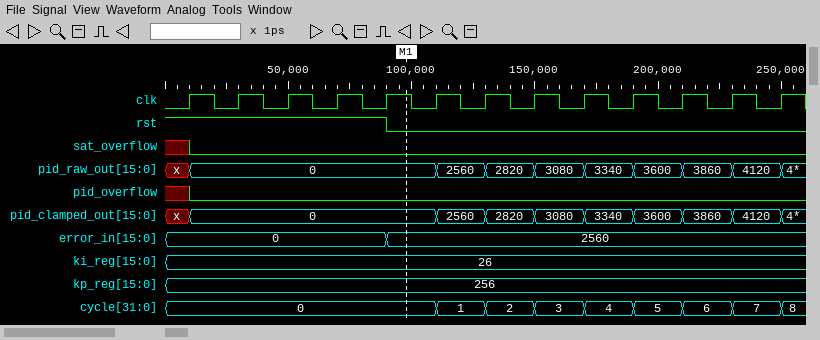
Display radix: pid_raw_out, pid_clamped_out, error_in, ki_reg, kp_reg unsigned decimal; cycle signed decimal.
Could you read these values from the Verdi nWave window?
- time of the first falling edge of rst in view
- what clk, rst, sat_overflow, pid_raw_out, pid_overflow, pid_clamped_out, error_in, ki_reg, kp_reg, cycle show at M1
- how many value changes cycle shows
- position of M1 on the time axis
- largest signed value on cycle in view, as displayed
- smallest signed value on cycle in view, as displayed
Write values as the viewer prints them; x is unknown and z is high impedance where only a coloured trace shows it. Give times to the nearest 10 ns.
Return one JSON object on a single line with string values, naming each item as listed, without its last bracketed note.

{"time of the first falling edge of rst in view": "90 ns", "what clk, rst, sat_overflow, pid_raw_out, pid_overflow, pid_clamped_out, error_in, ki_reg, kp_reg, cycle show at M1": "clk=1, rst=0, sat_overflow=0, pid_raw_out=0, pid_overflow=0, pid_clamped_out=0, error_in=2560, ki_reg=26, kp_reg=256, cycle=0", "how many value changes cycle shows": "8", "position of M1 on the time axis": "100 ns", "largest signed value on cycle in view, as displayed": "8", "smallest signed value on cycle in view, as displayed": "0"}
